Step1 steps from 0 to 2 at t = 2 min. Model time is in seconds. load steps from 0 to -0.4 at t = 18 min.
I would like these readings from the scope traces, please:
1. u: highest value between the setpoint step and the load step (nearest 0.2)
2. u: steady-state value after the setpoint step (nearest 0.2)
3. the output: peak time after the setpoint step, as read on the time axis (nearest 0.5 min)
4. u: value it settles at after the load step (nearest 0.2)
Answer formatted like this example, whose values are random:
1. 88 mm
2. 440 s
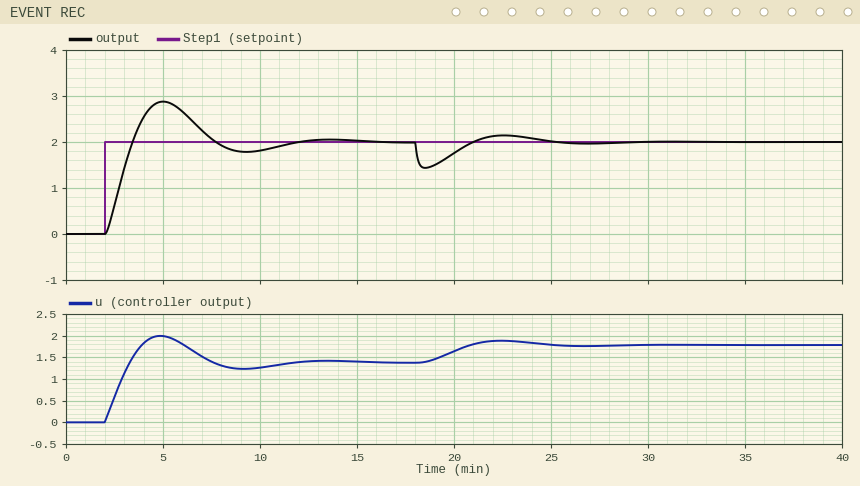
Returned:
1. 2.0
2. 1.4
3. 5.0 min
4. 1.8
